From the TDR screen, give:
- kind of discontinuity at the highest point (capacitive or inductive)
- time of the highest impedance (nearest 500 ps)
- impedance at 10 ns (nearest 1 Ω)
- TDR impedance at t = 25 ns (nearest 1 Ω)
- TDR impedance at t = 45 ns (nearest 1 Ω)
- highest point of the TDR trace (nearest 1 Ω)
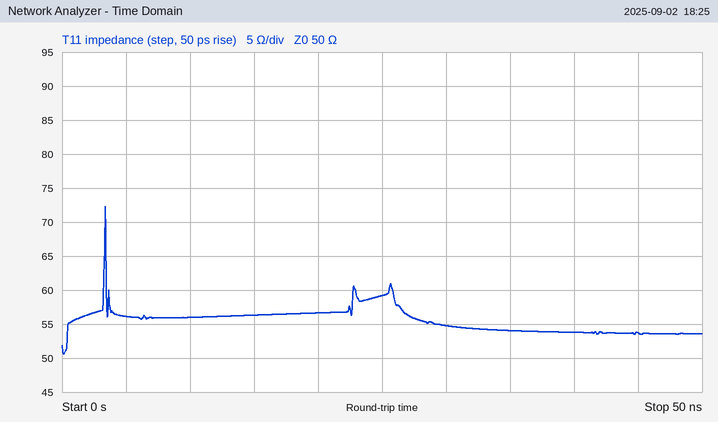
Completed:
inductive
3.5 ns
56 Ω
59 Ω
54 Ω
72 Ω
